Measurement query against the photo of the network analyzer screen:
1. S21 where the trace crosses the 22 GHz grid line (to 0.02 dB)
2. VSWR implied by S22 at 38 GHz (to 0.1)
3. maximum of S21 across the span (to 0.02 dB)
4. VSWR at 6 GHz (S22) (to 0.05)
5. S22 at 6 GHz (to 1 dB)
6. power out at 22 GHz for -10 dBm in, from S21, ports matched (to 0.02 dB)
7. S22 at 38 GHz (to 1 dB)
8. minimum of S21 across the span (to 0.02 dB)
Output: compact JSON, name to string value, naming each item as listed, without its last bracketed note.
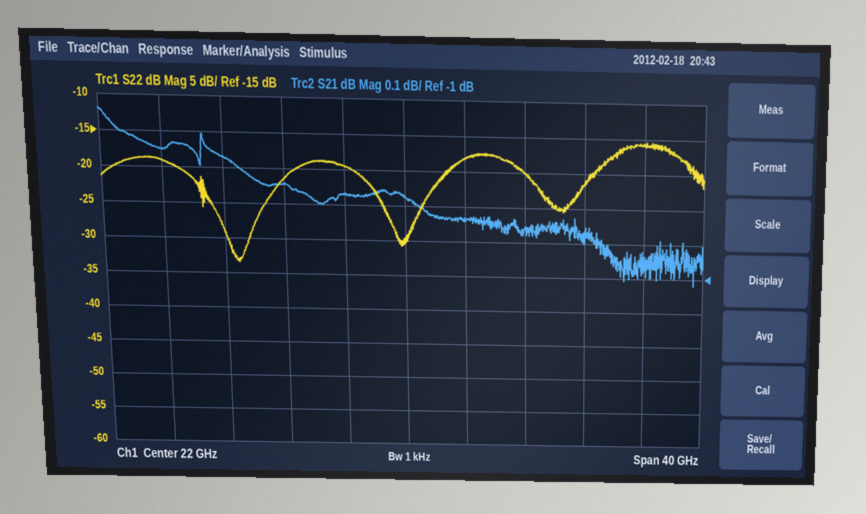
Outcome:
{"S21 where the trace crosses the 22 GHz grid line": "-0.78 dB", "VSWR implied by S22 at 38 GHz": "1.4", "maximum of S21 across the span": "-0.54 dB", "VSWR at 6 GHz (S22)": "1.25", "S22 at 6 GHz": "-19 dB", "power out at 22 GHz for -10 dBm in, from S21, ports matched": "-10.78 dBm", "S22 at 38 GHz": "-16 dB", "minimum of S21 across the span": "-1.02 dB"}
